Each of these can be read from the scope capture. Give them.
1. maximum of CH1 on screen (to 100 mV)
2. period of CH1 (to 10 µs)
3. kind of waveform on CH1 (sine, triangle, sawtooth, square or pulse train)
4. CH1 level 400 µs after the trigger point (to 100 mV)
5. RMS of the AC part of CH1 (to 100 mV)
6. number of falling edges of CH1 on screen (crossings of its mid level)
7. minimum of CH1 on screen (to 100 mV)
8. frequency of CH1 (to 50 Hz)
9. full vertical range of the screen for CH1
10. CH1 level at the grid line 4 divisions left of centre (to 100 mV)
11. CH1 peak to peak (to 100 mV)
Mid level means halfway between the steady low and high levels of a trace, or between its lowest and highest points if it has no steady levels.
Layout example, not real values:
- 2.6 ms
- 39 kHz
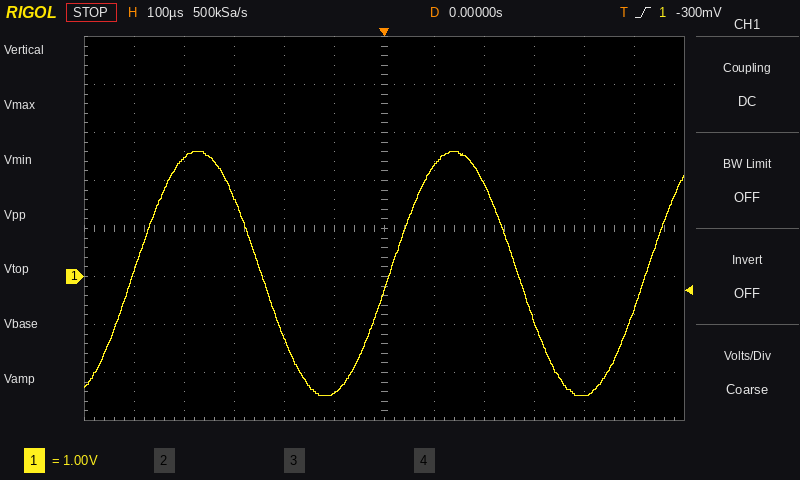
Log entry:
- 2.6 V
- 510 µs
- sine
- -2.5 V
- 1.8 V
- 2
- -2.5 V
- 1.95 kHz
- 8 V
- 2.5 V
- 5.1 V
